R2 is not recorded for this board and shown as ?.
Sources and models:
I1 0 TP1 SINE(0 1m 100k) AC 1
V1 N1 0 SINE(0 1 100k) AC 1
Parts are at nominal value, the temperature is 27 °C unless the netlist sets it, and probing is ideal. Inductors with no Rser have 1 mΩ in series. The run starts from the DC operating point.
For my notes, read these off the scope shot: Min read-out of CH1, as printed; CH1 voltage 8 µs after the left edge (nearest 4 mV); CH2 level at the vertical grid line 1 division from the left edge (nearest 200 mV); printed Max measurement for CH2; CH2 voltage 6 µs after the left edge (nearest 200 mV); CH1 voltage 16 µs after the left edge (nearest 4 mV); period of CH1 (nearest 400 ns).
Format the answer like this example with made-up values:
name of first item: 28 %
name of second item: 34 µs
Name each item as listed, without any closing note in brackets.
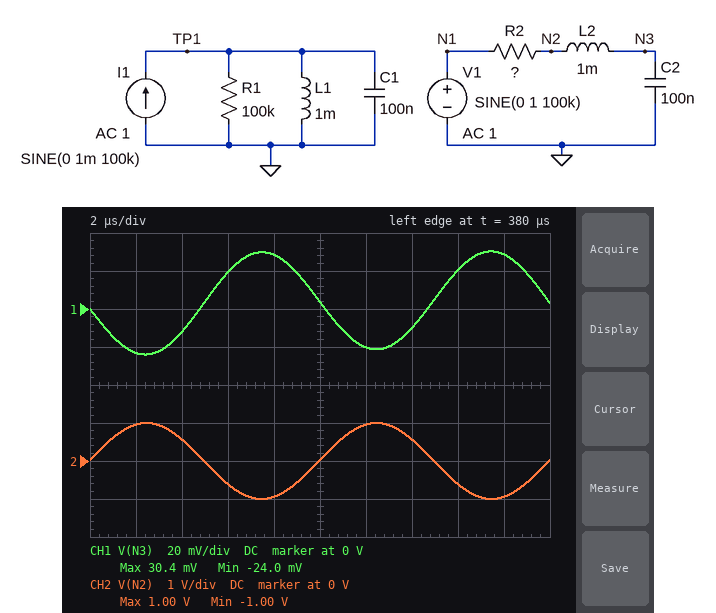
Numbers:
Min read-out of CH1, as printed: -24.0 mV
CH1 voltage 8 µs after the left edge: 28 mV
CH2 level at the vertical grid line 1 division from the left edge: 1.0 V
printed Max measurement for CH2: 1.00 V
CH2 voltage 6 µs after the left edge: -600 mV
CH1 voltage 16 µs after the left edge: 20 mV
period of CH1: 10.0 µs
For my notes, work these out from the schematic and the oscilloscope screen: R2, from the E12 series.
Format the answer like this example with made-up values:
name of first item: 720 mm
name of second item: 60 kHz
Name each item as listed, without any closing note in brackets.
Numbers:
R2, from the E12 series: 18 Ω
